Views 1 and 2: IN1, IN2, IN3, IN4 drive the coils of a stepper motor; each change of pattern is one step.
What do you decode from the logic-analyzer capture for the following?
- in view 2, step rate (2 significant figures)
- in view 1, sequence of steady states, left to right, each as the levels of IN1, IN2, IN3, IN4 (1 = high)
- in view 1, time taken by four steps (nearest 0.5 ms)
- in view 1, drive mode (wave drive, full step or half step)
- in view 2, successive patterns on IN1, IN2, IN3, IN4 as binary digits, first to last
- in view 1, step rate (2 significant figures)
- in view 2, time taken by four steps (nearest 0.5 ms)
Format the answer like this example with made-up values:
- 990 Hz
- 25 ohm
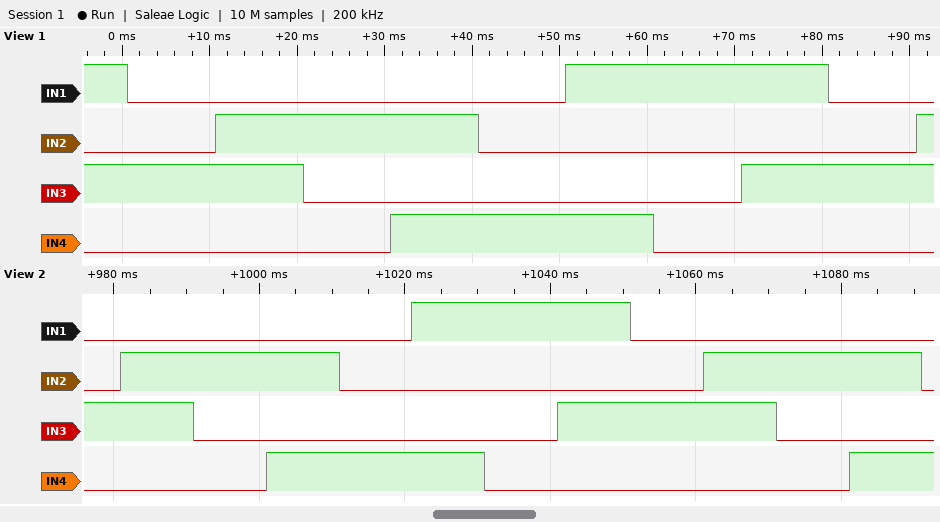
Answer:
- 100 steps/s
- 1010 0010 0110 0100 0101 0001 1001 1000 1010 0010 0110
- 40.0 ms
- half step
- 0010 0110 0100 0101 0001 1001 1000 1010 0010 0110 0100 0101 0001
- 100 steps/s
- 40.0 ms
